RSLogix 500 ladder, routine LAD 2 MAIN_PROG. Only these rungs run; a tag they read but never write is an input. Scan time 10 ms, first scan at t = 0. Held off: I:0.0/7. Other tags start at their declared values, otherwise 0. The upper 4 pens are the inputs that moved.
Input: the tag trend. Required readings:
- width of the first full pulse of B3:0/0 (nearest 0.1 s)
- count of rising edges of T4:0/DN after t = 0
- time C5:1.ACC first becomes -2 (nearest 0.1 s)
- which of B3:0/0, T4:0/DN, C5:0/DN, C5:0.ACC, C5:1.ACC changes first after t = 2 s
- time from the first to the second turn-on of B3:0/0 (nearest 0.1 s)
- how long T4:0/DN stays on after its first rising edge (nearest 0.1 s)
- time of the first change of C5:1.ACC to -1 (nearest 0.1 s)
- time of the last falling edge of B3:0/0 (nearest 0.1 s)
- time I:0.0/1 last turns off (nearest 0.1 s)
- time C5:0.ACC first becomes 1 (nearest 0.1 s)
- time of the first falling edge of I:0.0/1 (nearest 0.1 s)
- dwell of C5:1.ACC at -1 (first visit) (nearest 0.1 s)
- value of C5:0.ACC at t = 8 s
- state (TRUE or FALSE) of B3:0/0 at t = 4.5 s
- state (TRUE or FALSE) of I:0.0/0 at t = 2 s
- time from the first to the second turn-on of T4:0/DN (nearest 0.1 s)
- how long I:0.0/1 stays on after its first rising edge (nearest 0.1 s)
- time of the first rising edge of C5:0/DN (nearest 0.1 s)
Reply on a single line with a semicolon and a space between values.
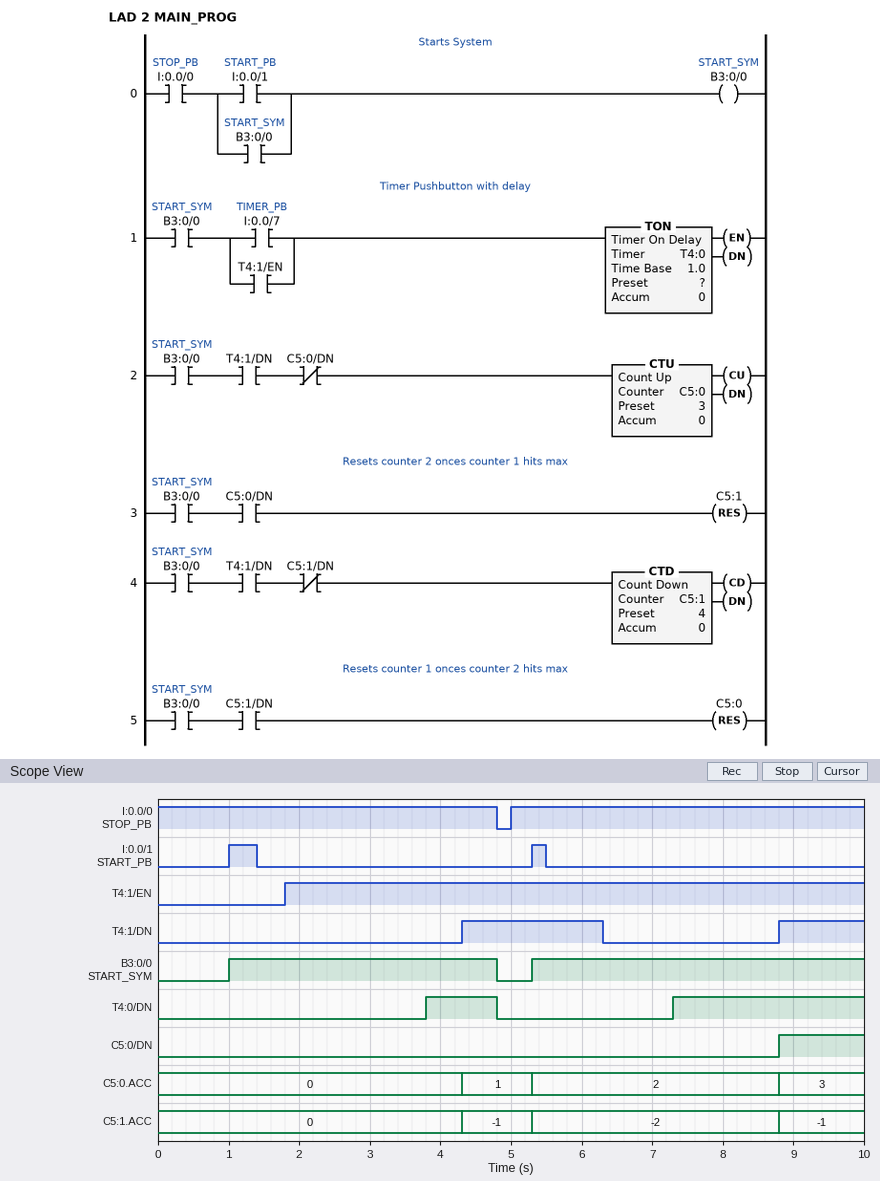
3.8 s; 2; 5.3 s; T4:0/DN; 4.3 s; 1.0 s; 4.3 s; 4.8 s; 5.5 s; 4.3 s; 1.4 s; 1.0 s; 2; TRUE; TRUE; 3.5 s; 0.4 s; 8.8 s
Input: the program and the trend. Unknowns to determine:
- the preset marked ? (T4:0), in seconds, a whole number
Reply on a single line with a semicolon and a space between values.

2 s
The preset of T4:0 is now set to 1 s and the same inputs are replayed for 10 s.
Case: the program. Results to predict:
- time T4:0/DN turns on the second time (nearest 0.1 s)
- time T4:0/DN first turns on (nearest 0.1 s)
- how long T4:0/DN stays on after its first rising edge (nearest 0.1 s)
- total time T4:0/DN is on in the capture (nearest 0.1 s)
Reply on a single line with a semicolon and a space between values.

6.3 s; 2.8 s; 2.0 s; 5.7 s
